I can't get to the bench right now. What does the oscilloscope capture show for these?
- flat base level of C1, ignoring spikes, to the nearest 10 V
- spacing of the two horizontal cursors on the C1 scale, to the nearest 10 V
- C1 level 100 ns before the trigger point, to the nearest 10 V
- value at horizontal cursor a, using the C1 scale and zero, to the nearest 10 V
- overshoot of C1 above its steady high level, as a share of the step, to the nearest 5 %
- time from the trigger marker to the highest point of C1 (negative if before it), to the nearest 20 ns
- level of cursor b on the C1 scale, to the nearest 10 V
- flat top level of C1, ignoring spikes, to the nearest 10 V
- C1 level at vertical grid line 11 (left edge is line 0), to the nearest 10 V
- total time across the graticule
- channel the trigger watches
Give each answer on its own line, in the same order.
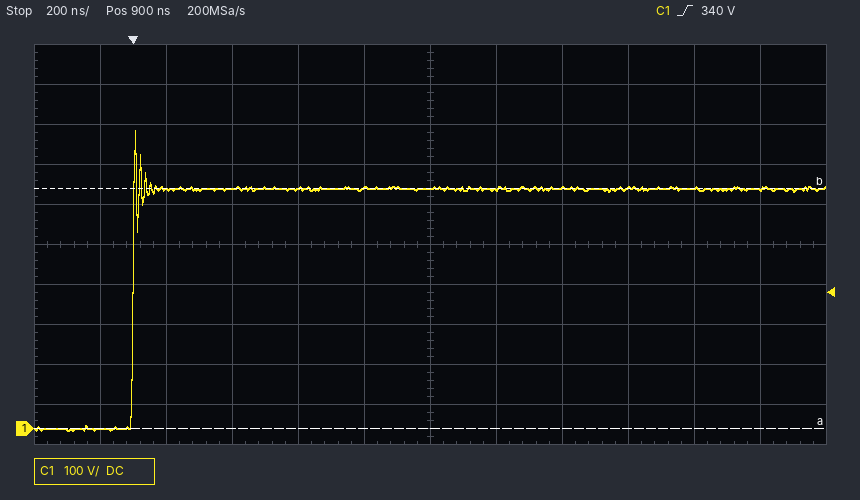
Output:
0 V
600 V
0 V
0 V
25 %
0 ns
600 V
600 V
600 V
2.4 µs
C1
